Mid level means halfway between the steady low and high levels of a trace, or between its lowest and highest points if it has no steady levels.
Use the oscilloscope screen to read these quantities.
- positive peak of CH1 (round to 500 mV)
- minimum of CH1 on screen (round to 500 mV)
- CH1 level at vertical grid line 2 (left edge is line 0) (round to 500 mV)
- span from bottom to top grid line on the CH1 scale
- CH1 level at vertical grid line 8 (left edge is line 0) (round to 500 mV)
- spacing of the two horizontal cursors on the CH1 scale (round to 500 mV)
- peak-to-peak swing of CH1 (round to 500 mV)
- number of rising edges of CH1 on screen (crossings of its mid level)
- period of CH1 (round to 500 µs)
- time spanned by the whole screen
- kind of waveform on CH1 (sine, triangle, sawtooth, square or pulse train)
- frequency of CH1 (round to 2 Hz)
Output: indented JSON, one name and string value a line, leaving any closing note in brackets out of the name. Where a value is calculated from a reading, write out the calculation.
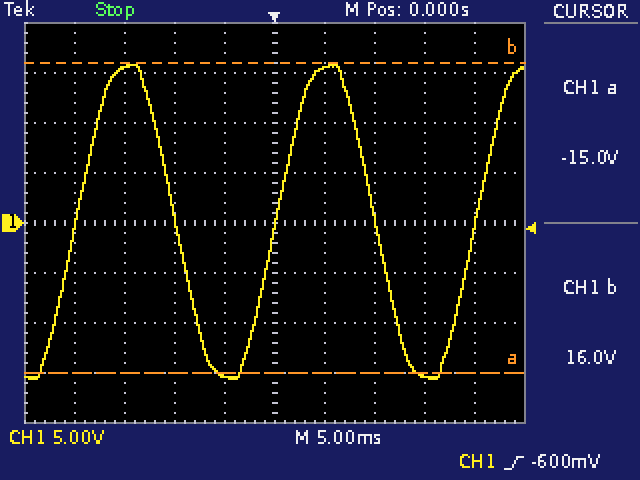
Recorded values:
{
  "positive peak of CH1": "16.0 V",
  "minimum of CH1 on screen": "-15.5 V",
  "CH1 level at vertical grid line 2 (left edge is line 0)": "15.5 V",
  "span from bottom to top grid line on the CH1 scale": "40 V",
  "CH1 level at vertical grid line 8 (left edge is line 0)": "-15.5 V",
  "spacing of the two horizontal cursors on the CH1 scale": "31.0 V",
  "peak-to-peak swing of CH1": "16.0 V − (-15.5 V) = 31.5 V",
  "number of rising edges of CH1 on screen": "3",
  "period of CH1": "20.0 ms",
  "time spanned by the whole screen": "50 ms",
  "kind of waveform on CH1": "sine",
  "frequency of CH1": "1 / 20.0 ms ≈ 50 Hz"
}
